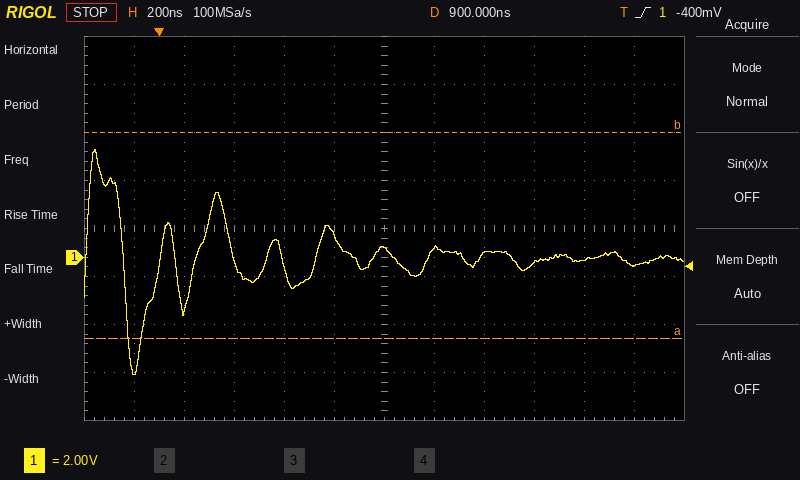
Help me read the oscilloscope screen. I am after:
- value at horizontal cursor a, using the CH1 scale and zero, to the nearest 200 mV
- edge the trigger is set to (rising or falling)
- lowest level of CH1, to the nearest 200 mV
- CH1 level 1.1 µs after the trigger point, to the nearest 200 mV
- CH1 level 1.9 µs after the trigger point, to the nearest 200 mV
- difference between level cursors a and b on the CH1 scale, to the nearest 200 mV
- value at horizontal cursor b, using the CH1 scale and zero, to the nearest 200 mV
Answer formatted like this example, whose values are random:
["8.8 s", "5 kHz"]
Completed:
["-3.4 V", "rising", "-4.8 V", "400 mV", "-400 mV", "8.6 V", "5.2 V"]
